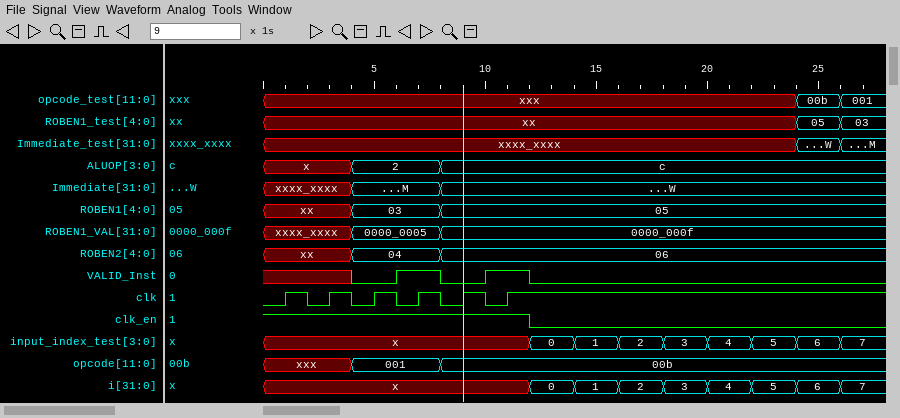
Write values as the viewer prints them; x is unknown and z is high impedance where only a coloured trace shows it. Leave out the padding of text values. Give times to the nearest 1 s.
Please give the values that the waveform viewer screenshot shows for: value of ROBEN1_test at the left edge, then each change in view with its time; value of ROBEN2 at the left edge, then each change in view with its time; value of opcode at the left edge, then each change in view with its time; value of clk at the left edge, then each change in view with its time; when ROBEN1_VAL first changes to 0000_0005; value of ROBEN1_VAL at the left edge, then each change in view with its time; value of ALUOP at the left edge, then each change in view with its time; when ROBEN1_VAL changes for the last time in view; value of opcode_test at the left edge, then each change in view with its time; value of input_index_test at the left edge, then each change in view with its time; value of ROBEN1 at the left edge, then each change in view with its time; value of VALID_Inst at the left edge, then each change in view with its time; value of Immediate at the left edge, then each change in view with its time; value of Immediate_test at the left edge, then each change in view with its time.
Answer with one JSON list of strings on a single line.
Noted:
["xx, 05 at 24 s, 03 at 26 s", "xx, 04 at 4 s, 06 at 8 s", "xxx, 001 at 4 s, 00b at 8 s", "0, 1 at 1 s, 0 at 2 s, 1 at 3 s, 0 at 4 s, 1 at 5 s, 0 at 6 s, 1 at 7 s, 0 at 8 s, 1 at 9 s, 0 at 10 s, 1 at 11 s", "4 s", "xxxx_xxxx, 0000_0005 at 4 s, 0000_000f at 8 s", "x, 2 at 4 s, c at 8 s", "8 s", "xxx, 00b at 24 s, 001 at 26 s", "x, 0 at 12 s, 1 at 14 s, 2 at 16 s, 3 at 18 s, 4 at 20 s, 5 at 22 s, 6 at 24 s, 7 at 26 s", "xx, 03 at 4 s, 05 at 8 s", "x, 0 at 4 s, 1 at 6 s, 0 at 8 s, 1 at 10 s, 0 at 12 s", "xxxx_xxxx, M at 4 s, W at 8 s", "xxxx_xxxx, W at 24 s, M at 26 s"]
